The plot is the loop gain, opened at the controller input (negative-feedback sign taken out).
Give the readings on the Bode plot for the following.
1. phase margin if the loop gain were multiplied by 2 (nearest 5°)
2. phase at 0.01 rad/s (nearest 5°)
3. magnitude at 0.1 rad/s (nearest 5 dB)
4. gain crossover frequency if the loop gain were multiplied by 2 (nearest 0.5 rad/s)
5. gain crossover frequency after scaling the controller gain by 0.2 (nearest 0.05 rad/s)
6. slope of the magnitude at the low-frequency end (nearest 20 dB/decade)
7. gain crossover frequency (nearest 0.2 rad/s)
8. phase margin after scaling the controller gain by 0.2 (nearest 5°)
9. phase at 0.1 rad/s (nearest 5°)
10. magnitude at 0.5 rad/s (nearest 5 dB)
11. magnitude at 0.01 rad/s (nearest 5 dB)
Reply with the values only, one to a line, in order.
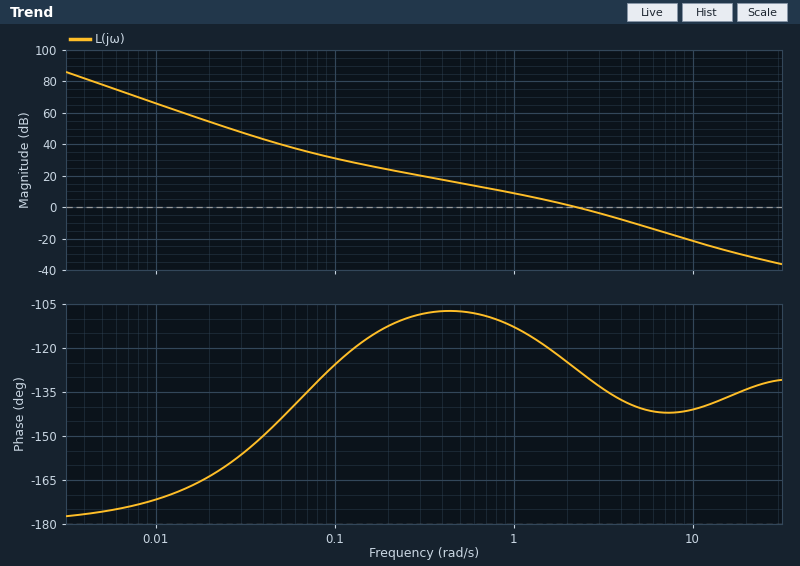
45°
-170°
30 dB
3.5 rad/s
0.60 rad/s
-40 dB/decade
2.2 rad/s
70°
-125°
15 dB
65 dB
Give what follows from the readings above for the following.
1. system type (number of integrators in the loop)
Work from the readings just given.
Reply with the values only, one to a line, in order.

2
